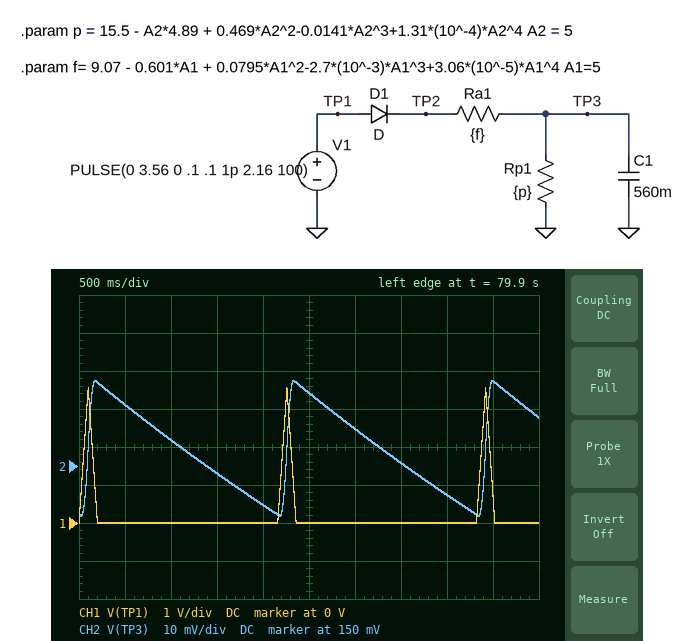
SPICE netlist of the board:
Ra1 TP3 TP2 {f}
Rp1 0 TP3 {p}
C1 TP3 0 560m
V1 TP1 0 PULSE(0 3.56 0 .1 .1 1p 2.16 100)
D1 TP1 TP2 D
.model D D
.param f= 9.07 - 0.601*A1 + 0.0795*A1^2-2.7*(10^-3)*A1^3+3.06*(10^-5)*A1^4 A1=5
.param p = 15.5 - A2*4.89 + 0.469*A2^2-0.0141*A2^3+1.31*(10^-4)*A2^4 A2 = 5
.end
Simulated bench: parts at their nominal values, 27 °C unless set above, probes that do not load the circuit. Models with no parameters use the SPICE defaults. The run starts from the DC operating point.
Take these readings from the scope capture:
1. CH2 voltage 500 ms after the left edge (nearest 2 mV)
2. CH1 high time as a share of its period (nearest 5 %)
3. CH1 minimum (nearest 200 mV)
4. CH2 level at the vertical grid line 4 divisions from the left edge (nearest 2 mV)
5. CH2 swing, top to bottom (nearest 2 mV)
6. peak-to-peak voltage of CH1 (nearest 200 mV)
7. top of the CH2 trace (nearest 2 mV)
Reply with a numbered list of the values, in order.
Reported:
1. 166 mV
2. 5 %
3. 0 V
4. 140 mV
5. 36 mV
6. 3.6 V
7. 172 mV
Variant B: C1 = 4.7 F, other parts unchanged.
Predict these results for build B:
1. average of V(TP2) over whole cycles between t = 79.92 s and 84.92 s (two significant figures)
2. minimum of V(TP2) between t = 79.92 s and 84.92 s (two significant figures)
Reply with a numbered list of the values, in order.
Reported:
1. 200 mV
2. 110 mV
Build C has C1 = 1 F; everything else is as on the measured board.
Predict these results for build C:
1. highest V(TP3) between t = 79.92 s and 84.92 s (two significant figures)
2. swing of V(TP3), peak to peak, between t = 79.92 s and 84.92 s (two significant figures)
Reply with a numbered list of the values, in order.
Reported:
1. 160 mV
2. 20 mV
